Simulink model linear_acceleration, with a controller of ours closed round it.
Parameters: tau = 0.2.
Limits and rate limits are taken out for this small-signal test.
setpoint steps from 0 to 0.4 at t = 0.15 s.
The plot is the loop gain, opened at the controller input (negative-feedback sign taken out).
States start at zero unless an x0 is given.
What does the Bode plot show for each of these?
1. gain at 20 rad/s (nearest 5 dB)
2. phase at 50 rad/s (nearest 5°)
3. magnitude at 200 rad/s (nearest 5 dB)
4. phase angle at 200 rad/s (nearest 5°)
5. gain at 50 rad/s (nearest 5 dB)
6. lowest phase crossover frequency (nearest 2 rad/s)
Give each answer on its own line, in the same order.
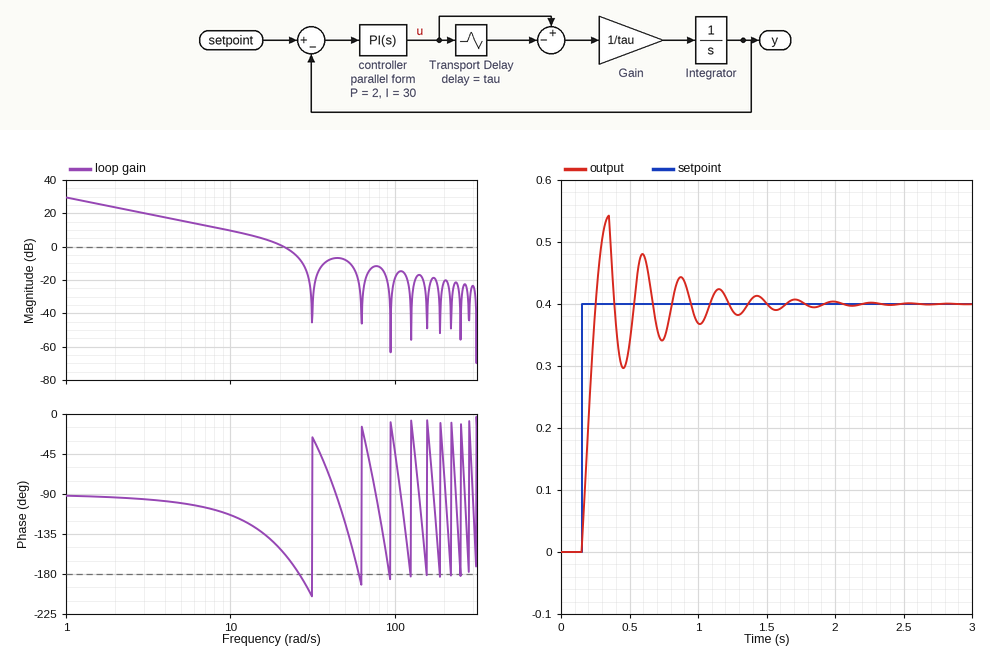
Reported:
0 dB
-125°
-20 dB
-70°
-10 dB
26 rad/s
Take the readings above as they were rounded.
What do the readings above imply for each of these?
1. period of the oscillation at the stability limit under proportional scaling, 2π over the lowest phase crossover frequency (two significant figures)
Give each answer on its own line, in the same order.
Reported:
0.24 s
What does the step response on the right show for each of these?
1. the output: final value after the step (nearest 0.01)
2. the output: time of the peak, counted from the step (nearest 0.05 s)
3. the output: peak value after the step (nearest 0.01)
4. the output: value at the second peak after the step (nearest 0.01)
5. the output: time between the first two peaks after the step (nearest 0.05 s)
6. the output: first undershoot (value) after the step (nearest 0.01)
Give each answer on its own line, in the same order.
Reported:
0.40
0.20 s
0.54
0.48
0.25 s
0.30
